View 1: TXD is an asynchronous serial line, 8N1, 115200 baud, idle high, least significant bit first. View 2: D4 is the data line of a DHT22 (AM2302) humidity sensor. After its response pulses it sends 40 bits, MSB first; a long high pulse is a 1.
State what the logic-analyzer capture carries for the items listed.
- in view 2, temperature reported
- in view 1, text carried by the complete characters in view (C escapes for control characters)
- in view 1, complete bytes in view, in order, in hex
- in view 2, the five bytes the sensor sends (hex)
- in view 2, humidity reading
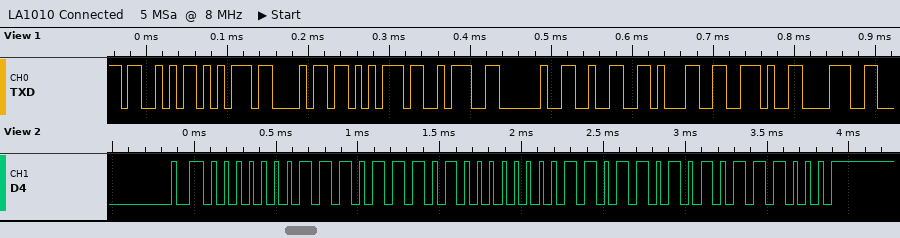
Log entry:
21.8 °C
"Suhu: 21.8"
53 75 68 75 3A 20 32 31 2E 38
01 DD 00 DA B8
47.7 %
